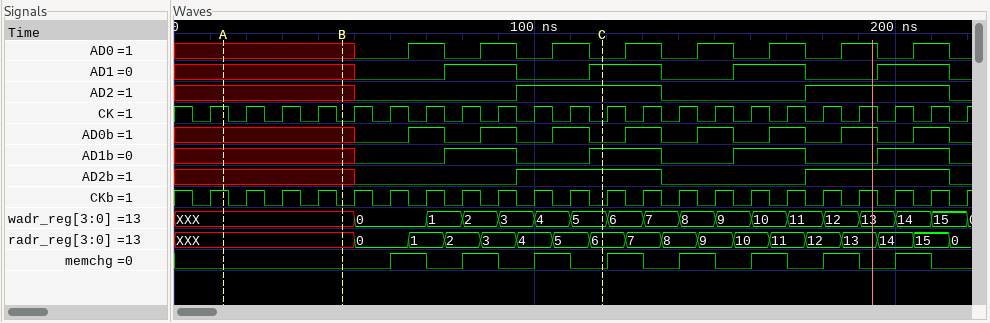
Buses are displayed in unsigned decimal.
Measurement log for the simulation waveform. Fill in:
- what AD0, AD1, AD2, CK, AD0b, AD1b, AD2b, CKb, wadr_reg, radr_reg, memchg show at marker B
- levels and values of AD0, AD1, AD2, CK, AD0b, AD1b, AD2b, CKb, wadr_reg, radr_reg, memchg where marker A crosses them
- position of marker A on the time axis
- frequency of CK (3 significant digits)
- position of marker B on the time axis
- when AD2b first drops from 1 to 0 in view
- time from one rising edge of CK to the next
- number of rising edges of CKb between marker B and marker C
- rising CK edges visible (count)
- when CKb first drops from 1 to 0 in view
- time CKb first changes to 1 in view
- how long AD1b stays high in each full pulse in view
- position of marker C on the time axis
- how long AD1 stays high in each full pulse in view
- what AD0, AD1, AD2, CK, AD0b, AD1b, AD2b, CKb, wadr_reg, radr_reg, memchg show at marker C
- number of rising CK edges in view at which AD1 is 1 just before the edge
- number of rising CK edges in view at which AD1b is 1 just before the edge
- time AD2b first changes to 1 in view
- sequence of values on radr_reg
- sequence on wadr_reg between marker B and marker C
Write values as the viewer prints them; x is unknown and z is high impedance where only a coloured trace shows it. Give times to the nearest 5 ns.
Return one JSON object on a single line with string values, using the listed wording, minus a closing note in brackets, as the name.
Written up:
{"what AD0, AD1, AD2, CK, AD0b, AD1b, AD2b, CKb, wadr_reg, radr_reg, memchg show at marker B": "AD0=x, AD1=x, AD2=x, CK=0, AD0b=x, AD1b=x, AD2b=x, CKb=0, wadr_reg=XXX, radr_reg=XXX, memchg=0", "levels and values of AD0, AD1, AD2, CK, AD0b, AD1b, AD2b, CKb, wadr_reg, radr_reg, memchg where marker A crosses them": "AD0=x, AD1=x, AD2=x, CK=1, AD0b=x, AD1b=x, AD2b=x, CKb=1, wadr_reg=XXX, radr_reg=XXX, memchg=0", "position of marker A on the time axis": "15 ns", "frequency of CK": "100 MHz", "position of marker B on the time axis": "45 ns", "when AD2b first drops from 1 to 0 in view": "135 ns", "time from one rising edge of CK to the next": "10 ns", "number of rising edges of CKb between marker B and marker C": "7", "rising CK edges visible": "22", "when CKb first drops from 1 to 0 in view": "5 ns", "time CKb first changes to 1 in view": "10 ns", "how long AD1b stays high in each full pulse in view": "20 ns, 20 ns, 20 ns, 20 ns", "position of marker C on the time axis": "120 ns", "how long AD1 stays high in each full pulse in view": "20 ns, 20 ns, 20 ns, 20 ns", "what AD0, AD1, AD2, CK, AD0b, AD1b, AD2b, CKb, wadr_reg, radr_reg, memchg show at marker C": "AD0=0, AD1=1, AD2=1, CK=0, AD0b=0, AD1b=1, AD2b=1, CKb=0, wadr_reg=5, radr_reg=6, memchg=0", "number of rising CK edges in view at which AD1 is 1 just before the edge": "8", "number of rising CK edges in view at which AD1b is 1 just before the edge": "8", "time AD2b first changes to 1 in view": "95 ns", "sequence of values on radr_reg": "XXX, 0, 1, 2, 3, 4, 5, 6, 7, 8, 9, 10, 11, 12, 13, 14, 15, 0", "sequence on wadr_reg between marker B and marker C": "XXX, 0, 1, 2, 3, 4, 5"}
